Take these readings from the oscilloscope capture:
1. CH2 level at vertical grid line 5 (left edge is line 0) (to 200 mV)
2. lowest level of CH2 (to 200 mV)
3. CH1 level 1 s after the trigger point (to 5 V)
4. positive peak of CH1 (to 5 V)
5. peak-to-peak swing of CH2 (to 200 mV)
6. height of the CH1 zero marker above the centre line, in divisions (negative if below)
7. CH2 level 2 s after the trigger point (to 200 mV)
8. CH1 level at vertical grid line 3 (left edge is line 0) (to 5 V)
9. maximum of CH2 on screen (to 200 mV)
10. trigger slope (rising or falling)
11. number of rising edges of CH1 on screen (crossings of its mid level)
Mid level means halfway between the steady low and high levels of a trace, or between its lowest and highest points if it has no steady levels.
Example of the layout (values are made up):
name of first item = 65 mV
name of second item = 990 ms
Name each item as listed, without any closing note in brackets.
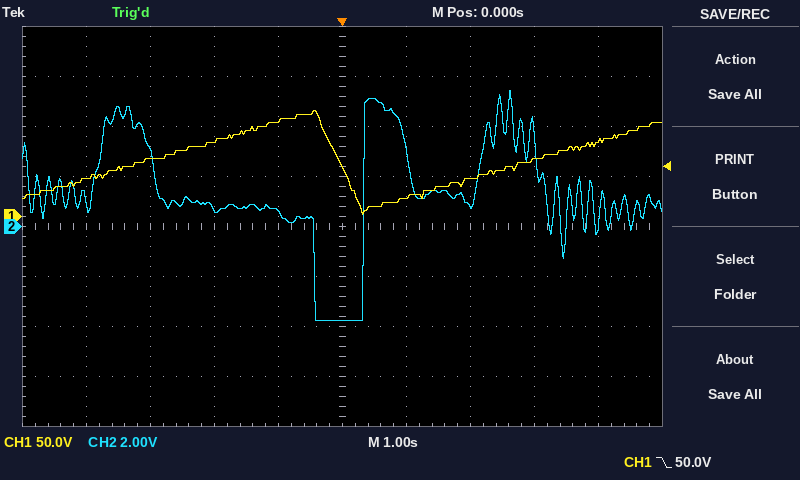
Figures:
CH2 level at vertical grid line 5 (left edge is line 0) = -3.8 V
lowest level of CH2 = -3.8 V
CH1 level 1 s after the trigger point = 20 V
positive peak of CH1 = 105 V
peak-to-peak swing of CH2 = 9.2 V
height of the CH1 zero marker above the centre line, in divisions = +0.2 div
CH2 level 2 s after the trigger point = 800 mV
CH1 level at vertical grid line 3 (left edge is line 0) = 75 V
maximum of CH2 on screen = 5.4 V
trigger slope = falling
number of rising edges of CH1 on screen = 2
